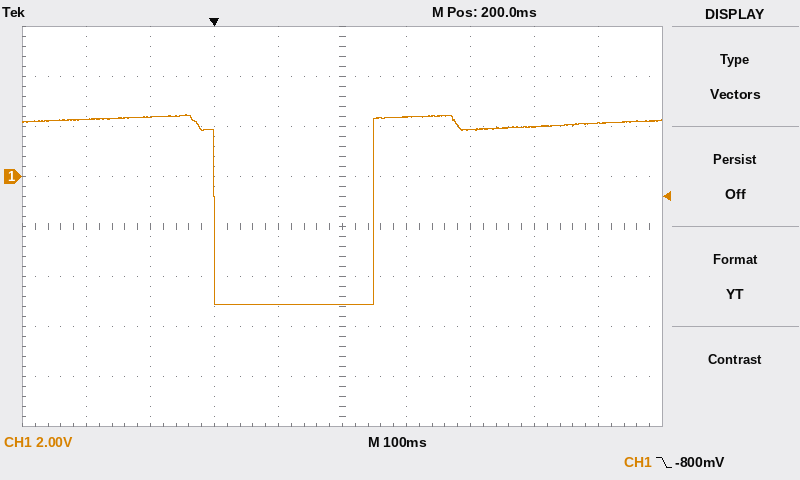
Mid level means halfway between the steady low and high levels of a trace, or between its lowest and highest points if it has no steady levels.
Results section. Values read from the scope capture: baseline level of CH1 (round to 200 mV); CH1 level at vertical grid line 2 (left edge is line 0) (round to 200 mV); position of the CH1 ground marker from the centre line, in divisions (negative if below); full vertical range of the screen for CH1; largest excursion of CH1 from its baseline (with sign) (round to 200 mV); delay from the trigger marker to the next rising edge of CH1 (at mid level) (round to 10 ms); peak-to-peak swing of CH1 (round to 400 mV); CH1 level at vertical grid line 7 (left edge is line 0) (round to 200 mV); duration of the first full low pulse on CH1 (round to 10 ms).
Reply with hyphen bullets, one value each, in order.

- 2.2 V
- 2.4 V
- +1.0 div
- 16 V
- -7.4 V
- 250 ms
- 7.6 V
- 1.8 V
- 250 ms
